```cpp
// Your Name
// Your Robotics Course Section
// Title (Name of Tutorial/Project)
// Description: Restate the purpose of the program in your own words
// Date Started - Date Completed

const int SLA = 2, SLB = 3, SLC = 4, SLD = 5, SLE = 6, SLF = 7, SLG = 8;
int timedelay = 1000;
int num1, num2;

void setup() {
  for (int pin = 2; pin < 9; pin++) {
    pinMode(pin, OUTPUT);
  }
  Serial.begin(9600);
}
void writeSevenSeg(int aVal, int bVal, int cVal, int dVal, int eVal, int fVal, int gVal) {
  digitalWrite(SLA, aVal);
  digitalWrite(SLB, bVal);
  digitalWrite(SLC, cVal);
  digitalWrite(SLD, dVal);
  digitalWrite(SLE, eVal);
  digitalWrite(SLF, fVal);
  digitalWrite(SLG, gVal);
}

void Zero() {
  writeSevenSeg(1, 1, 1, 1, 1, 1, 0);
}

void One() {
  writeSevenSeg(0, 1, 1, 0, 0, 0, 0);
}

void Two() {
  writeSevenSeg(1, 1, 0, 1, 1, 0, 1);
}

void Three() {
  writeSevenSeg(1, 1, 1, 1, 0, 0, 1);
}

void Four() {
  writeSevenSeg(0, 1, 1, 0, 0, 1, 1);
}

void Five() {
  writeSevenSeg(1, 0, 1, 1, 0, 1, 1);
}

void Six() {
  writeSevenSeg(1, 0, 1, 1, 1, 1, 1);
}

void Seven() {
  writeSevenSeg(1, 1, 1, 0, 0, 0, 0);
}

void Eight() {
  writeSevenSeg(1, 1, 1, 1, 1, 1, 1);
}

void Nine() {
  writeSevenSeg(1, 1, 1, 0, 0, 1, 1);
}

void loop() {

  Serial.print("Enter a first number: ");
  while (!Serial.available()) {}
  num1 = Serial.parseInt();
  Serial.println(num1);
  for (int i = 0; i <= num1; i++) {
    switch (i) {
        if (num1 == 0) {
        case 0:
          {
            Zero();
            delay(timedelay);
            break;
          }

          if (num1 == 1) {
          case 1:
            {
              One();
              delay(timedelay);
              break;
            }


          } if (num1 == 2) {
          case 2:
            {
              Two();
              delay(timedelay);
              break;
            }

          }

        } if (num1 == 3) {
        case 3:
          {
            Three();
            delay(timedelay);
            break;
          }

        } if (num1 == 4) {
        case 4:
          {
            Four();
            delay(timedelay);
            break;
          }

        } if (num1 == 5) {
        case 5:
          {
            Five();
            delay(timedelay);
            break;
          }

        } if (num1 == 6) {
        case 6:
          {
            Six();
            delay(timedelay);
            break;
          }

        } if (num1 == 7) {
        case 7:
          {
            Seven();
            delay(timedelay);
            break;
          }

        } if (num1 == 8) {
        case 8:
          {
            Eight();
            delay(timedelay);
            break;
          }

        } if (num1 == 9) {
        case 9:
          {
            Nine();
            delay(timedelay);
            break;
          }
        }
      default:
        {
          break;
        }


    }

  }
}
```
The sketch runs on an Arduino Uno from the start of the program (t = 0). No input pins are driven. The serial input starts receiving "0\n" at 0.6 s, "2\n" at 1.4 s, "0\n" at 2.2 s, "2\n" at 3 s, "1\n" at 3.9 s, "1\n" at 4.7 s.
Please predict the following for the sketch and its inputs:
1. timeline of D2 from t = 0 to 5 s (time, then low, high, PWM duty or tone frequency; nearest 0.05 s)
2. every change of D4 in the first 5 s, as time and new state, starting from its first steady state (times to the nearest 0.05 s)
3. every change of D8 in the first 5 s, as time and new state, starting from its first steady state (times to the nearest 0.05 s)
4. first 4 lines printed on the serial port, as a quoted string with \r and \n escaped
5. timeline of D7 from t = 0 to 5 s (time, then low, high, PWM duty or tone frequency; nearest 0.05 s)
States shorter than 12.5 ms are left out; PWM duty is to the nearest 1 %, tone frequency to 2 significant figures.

0 s low; 0.6 s high; 2.6 s low; 3.6 s high
0 s low; 0.6 s high; 3.6 s low; 4.6 s high
0 s low; 3.6 s high; 4.6 s low
"Enter a first number: 0\r\nEnter a first number: 2\r\nEnter a first number: 0\r\nEnter a first number: 2\r\n"
0 s low; 0.6 s high; 2.6 s low; 4.6 s high
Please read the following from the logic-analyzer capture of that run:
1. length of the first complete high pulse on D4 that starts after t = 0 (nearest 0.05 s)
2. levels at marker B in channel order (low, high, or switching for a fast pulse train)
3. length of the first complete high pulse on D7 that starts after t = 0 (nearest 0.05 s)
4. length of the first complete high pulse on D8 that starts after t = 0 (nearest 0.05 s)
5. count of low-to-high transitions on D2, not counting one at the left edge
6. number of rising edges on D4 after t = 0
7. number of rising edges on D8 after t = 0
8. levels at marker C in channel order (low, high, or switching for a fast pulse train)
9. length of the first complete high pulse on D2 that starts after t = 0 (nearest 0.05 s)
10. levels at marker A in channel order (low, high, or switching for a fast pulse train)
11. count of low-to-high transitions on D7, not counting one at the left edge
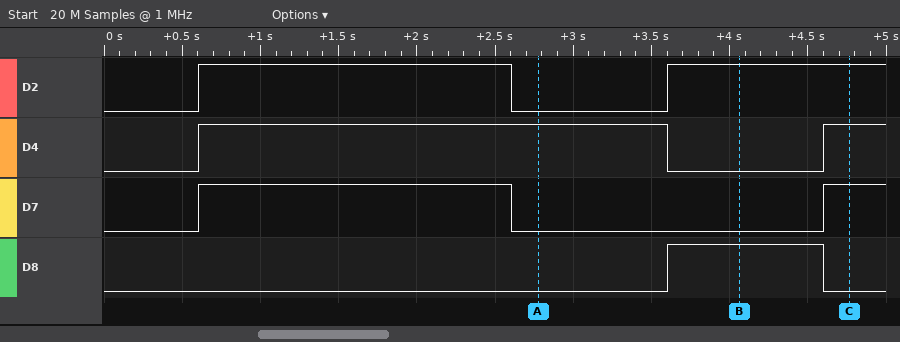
3.00 s
D2 high, D4 low, D7 low, D8 high
2.00 s
1.00 s
2
2
1
D2 high, D4 high, D7 high, D8 low
2.00 s
D2 low, D4 high, D7 low, D8 low
2
